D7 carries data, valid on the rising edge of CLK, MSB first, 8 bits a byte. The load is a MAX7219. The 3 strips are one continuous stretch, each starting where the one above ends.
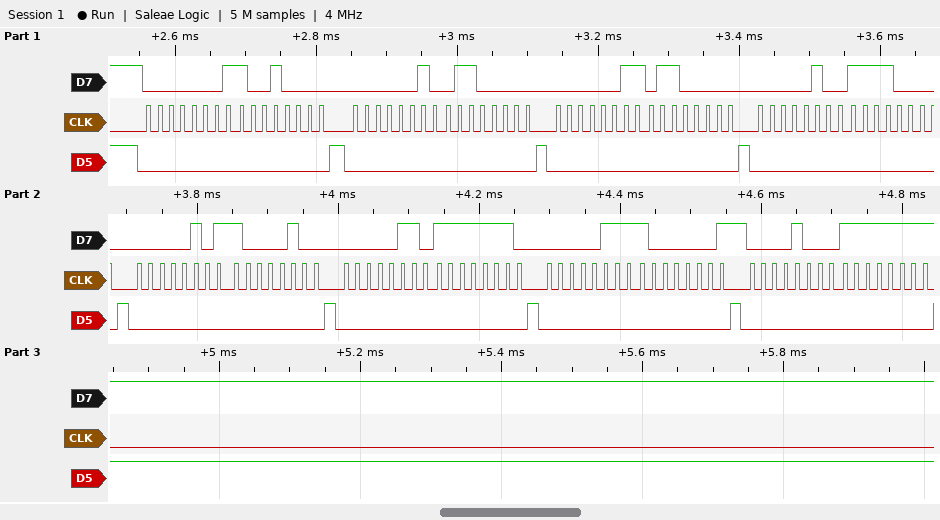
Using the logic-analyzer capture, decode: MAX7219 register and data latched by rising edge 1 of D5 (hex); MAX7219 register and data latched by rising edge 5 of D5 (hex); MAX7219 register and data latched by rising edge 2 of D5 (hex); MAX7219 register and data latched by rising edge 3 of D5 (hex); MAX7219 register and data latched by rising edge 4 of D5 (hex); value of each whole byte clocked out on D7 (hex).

register 0x1, data 0x90
register 0x5, data 0x84
register 0x2, data 0x60
register 0x3, data 0x60
register 0x4, data 0xF0
01 90 02 60 03 60 04 F0 05 84 06 FE 07 81 08 FF
